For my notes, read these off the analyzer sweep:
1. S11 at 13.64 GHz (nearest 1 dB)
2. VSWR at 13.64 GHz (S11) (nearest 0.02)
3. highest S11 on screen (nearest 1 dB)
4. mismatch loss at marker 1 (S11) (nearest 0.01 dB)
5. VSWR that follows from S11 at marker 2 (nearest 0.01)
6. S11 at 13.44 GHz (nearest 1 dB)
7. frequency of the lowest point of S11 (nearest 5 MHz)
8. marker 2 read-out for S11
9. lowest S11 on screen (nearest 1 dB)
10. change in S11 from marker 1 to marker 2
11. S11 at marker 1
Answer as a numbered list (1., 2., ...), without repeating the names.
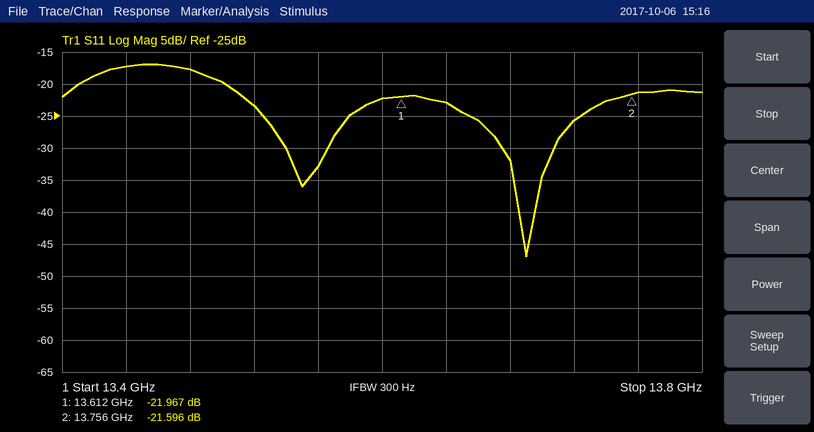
1. -23 dB
2. 1.16
3. -17 dB
4. 0.03 dB
5. 1.18
6. -17 dB
7. 13.690 GHz
8. -21.596 dB
9. -47 dB
10. 0.371 dB
11. -21.967 dB
